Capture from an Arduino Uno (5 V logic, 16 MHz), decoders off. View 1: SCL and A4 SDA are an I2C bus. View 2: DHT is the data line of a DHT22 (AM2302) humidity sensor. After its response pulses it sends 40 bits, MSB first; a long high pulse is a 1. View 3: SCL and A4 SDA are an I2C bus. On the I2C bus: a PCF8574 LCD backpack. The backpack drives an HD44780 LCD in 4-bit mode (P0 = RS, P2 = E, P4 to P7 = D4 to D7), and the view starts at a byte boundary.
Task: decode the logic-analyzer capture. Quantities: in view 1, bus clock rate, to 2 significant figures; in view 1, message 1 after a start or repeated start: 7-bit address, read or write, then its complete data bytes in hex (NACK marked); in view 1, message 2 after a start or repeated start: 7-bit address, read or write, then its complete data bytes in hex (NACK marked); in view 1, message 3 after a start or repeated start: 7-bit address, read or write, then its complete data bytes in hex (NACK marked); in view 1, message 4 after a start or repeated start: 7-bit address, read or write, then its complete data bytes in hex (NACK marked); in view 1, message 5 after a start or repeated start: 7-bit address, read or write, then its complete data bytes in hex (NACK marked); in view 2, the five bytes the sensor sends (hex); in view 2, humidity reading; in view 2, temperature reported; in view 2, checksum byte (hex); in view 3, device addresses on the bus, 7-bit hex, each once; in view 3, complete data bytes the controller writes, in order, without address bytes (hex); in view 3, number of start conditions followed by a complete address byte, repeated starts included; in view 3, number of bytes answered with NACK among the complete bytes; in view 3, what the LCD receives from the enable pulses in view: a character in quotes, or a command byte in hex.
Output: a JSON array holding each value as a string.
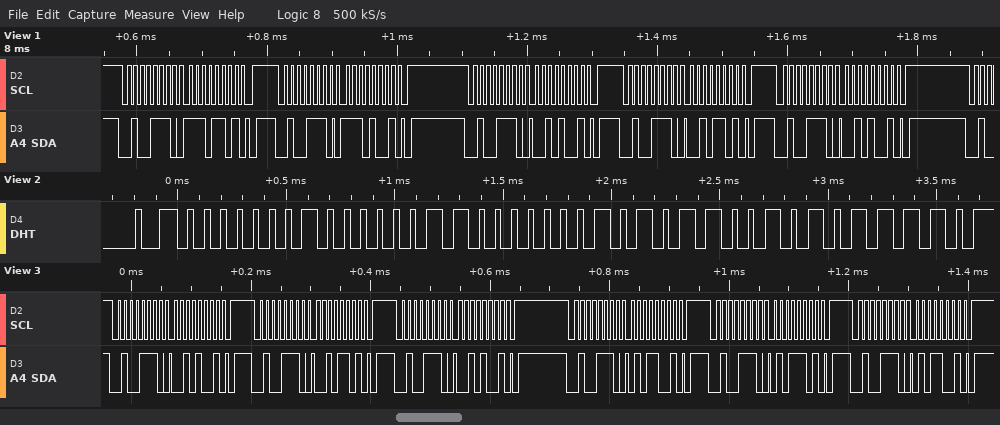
["100 kHz", "0x27 write: ED", "0x27 write: E9", "0x27 write: 29", "0x27 write: 2D", "0x27 write: 29", "01 03 01 59 5E", "25.9 %", "34.5 °C", "0x5E", "0x27", "29 2D 29 59 5D 59", "6", "0", "'%'"]
